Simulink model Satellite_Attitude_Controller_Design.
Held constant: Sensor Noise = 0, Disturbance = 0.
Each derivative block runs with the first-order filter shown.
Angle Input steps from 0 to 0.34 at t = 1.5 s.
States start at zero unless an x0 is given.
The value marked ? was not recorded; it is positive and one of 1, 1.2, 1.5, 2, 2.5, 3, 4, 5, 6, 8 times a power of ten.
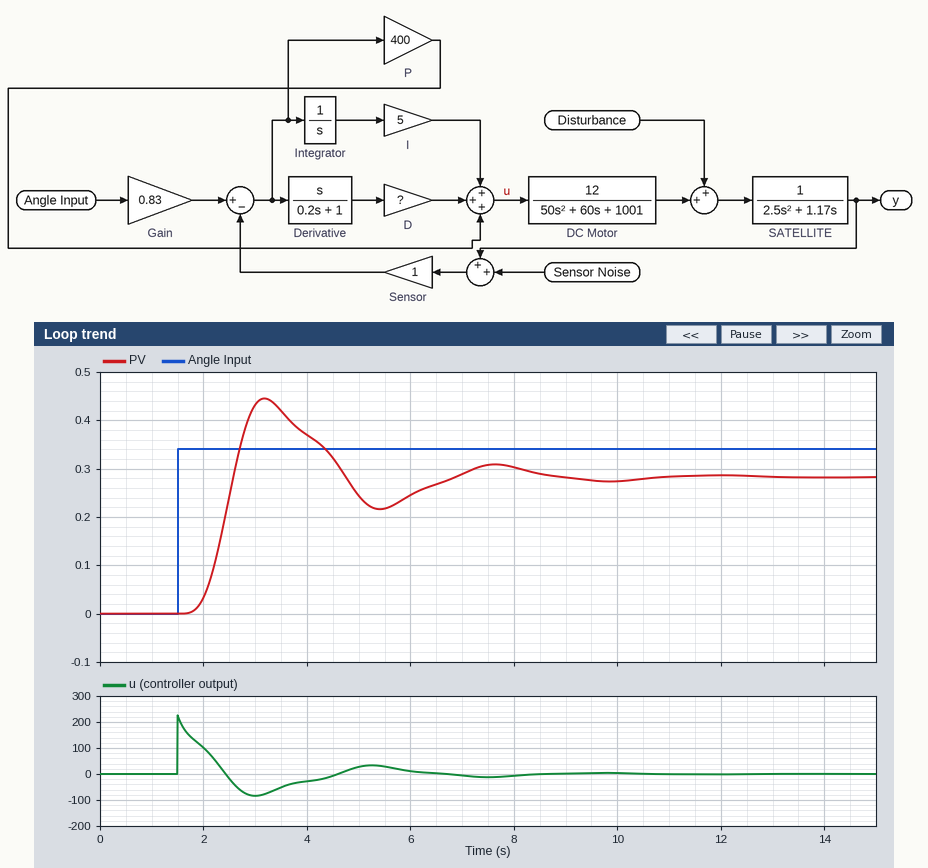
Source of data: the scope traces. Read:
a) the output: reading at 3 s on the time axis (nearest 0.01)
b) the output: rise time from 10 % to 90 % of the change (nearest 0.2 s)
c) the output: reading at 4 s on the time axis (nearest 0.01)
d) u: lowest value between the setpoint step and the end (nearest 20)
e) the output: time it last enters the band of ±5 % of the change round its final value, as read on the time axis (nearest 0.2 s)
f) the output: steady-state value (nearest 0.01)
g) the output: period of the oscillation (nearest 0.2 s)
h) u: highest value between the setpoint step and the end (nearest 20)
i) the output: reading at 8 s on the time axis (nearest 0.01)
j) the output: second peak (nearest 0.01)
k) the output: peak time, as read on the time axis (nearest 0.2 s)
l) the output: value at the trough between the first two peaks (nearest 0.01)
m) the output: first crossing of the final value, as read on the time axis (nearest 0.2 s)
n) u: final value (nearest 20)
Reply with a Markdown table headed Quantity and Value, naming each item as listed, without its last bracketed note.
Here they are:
| Quantity | Value |
|---|---|
| the output: reading at 3 s on the time axis | 0.43 |
| the output: rise time from 10 % to 90 % of the change | 0.6 s |
| the output: reading at 4 s on the time axis | 0.37 |
| u: lowest value between the setpoint step and the end | -80 |
| the output: time it last enters the band of ±5 % of the change round its final value, as read on the time axis | 8.2 s |
| the output: steady-state value | 0.28 |
| the output: period of the oscillation | 4.4 s |
| u: highest value between the setpoint step and the end | 220 |
| the output: reading at 8 s on the time axis | 0.30 |
| the output: second peak | 0.31 |
| the output: peak time, as read on the time axis | 3.2 s |
| the output: value at the trough between the first two peaks | 0.22 |
| the output: first crossing of the final value, as read on the time axis | 2.6 s |
| u: final value | 0 |
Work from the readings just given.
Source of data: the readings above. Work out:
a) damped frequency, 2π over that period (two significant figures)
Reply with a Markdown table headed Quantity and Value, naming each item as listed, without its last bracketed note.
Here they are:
| Quantity | Value |
|---|---|
| damped frequency, 2π over that period | 1.4 rad/s |
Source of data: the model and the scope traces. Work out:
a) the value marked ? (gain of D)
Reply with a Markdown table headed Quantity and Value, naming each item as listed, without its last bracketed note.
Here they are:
| Quantity | Value |
|---|---|
| the value marked ? | 80 |
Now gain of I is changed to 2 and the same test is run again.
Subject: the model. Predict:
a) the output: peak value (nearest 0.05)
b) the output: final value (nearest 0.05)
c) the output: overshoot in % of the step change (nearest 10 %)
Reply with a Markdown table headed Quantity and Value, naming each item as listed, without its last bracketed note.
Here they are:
| Quantity | Value |
|---|---|
| the output: peak value | 0.45 |
| the output: final value | 0.30 |
| the output: overshoot in % of the step change | 60 % |
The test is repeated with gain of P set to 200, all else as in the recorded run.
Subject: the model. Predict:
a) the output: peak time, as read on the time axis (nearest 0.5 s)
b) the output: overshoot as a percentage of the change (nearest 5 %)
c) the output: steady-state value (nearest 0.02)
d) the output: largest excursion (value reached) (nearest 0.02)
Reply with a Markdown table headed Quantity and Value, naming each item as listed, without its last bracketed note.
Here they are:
| Quantity | Value |
|---|---|
| the output: peak time, as read on the time axis | 4.5 s |
| the output: overshoot as a percentage of the change | 35 % |
| the output: steady-state value | 0.28 |
| the output: largest excursion (value reached) | 0.38 |
